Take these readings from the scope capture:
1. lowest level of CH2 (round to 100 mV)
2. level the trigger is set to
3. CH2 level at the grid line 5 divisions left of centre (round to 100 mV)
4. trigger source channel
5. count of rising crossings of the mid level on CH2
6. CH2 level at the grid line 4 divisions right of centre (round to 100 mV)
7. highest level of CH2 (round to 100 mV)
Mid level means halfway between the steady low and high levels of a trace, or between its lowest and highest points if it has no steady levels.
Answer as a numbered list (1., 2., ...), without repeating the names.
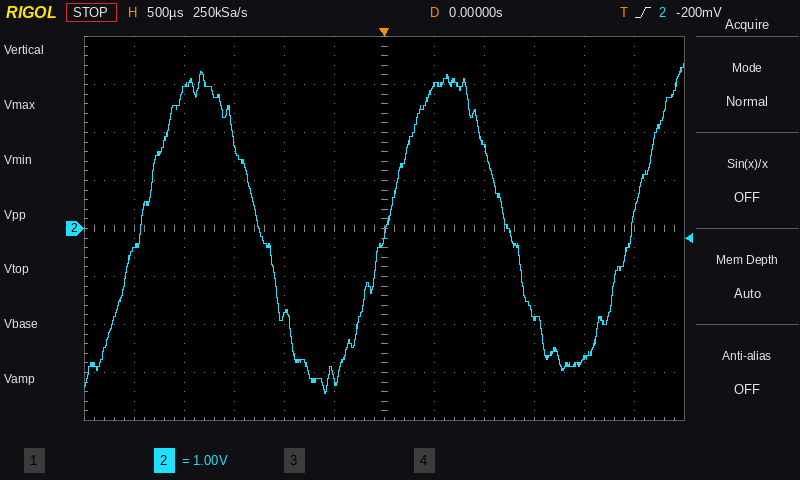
1. -3.4 V
2. -200 mV
3. -400 mV
4. CH2
5. 3
6. -2.7 V
7. 3.4 V
